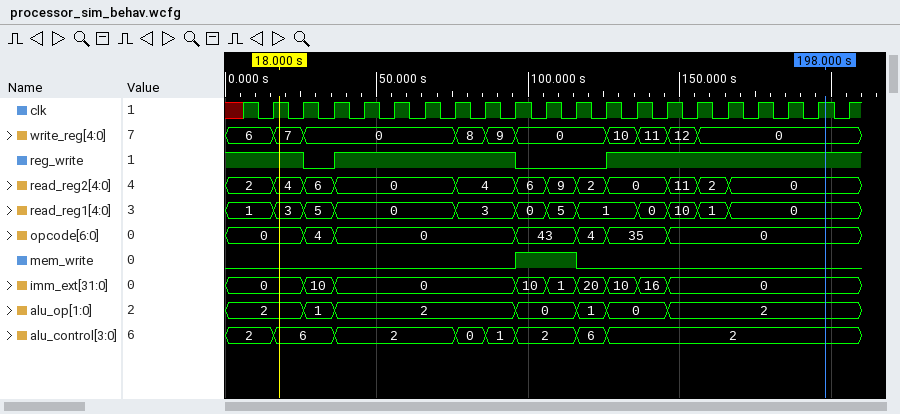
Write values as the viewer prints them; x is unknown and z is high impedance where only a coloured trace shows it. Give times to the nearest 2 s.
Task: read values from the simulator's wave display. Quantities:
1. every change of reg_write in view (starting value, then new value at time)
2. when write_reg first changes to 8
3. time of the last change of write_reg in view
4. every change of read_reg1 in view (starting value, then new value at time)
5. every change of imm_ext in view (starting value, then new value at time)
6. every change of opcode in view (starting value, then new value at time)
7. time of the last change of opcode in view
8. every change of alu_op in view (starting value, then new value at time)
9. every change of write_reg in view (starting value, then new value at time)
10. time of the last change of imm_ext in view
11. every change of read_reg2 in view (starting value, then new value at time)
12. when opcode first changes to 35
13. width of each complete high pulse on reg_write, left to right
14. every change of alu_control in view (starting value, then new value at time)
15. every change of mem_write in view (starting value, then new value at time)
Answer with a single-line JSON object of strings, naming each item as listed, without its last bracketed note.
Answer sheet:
{"every change of reg_write in view": "1, 0 at 26 s, 1 at 36 s, 0 at 96 s, 1 at 126 s", "when write_reg first changes to 8": "76 s", "time of the last change of write_reg in view": "156 s", "every change of read_reg1 in view": "1, 3 at 16 s, 5 at 26 s, 0 at 36 s, 3 at 76 s, 0 at 96 s, 5 at 106 s, 1 at 116 s, 0 at 136 s, 10 at 146 s, 1 at 156 s, 0 at 166 s", "every change of imm_ext in view": "0, 10 at 26 s, 0 at 36 s, 10 at 96 s, 1 at 106 s, 20 at 116 s, 10 at 126 s, 16 at 136 s, 0 at 146 s", "every change of opcode in view": "0, 4 at 26 s, 0 at 36 s, 43 at 96 s, 4 at 116 s, 35 at 126 s, 0 at 146 s", "time of the last change of opcode in view": "146 s", "every change of alu_op in view": "2, 1 at 26 s, 2 at 36 s, 0 at 96 s, 1 at 116 s, 0 at 126 s, 2 at 146 s", "every change of write_reg in view": "6, 7 at 16 s, 0 at 26 s, 8 at 76 s, 9 at 86 s, 0 at 96 s, 10 at 126 s, 11 at 136 s, 12 at 146 s, 0 at 156 s", "time of the last change of imm_ext in view": "146 s", "every change of read_reg2 in view": "2, 4 at 16 s, 6 at 26 s, 0 at 36 s, 4 at 76 s, 6 at 96 s, 9 at 106 s, 2 at 116 s, 0 at 126 s, 11 at 146 s, 2 at 156 s, 0 at 166 s", "when opcode first changes to 35": "126 s", "width of each complete high pulse on reg_write, left to right": "60 s", "every change of alu_control in view": "2, 6 at 16 s, 2 at 36 s, 0 at 76 s, 1 at 86 s, 2 at 96 s, 6 at 116 s, 2 at 126 s", "every change of mem_write in view": "0, 1 at 96 s, 0 at 116 s"}
